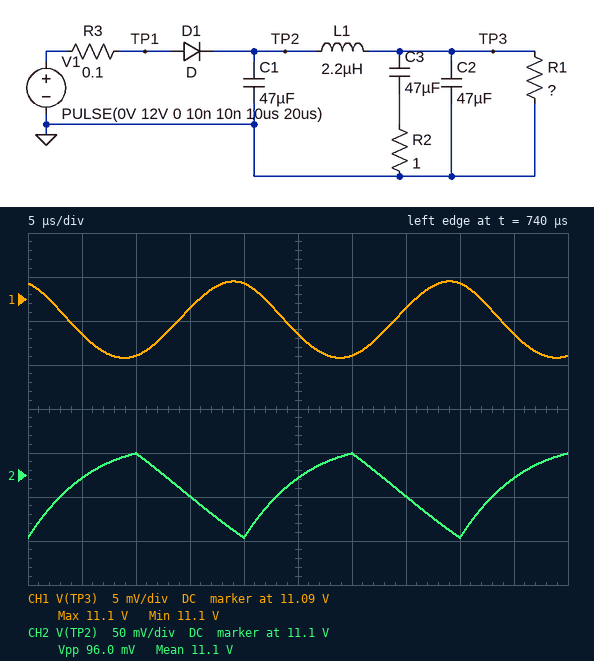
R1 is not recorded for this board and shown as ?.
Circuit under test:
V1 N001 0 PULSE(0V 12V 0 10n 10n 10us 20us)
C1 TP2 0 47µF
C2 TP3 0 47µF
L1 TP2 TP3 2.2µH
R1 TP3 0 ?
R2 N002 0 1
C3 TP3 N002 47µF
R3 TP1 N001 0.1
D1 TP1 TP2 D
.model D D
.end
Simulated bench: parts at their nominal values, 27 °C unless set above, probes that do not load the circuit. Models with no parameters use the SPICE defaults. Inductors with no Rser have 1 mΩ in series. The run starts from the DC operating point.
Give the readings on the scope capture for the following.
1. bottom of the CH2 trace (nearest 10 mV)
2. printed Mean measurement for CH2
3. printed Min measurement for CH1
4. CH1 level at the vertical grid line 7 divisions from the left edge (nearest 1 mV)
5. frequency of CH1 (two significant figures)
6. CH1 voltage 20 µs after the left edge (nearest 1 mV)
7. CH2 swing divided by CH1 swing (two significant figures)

11.03 V
11.1 V
11.1 V
11.084 V
50 kHz
11.087 V
11
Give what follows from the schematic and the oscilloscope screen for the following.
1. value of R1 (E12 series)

27 Ω
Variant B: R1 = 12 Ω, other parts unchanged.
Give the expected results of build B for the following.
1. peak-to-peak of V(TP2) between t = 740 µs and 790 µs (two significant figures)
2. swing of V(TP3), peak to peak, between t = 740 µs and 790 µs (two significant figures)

210 mV
19 mV
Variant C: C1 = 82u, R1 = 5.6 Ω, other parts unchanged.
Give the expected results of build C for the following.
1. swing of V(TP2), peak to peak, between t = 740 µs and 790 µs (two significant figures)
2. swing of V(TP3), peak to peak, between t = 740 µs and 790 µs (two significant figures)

250 mV
22 mV
